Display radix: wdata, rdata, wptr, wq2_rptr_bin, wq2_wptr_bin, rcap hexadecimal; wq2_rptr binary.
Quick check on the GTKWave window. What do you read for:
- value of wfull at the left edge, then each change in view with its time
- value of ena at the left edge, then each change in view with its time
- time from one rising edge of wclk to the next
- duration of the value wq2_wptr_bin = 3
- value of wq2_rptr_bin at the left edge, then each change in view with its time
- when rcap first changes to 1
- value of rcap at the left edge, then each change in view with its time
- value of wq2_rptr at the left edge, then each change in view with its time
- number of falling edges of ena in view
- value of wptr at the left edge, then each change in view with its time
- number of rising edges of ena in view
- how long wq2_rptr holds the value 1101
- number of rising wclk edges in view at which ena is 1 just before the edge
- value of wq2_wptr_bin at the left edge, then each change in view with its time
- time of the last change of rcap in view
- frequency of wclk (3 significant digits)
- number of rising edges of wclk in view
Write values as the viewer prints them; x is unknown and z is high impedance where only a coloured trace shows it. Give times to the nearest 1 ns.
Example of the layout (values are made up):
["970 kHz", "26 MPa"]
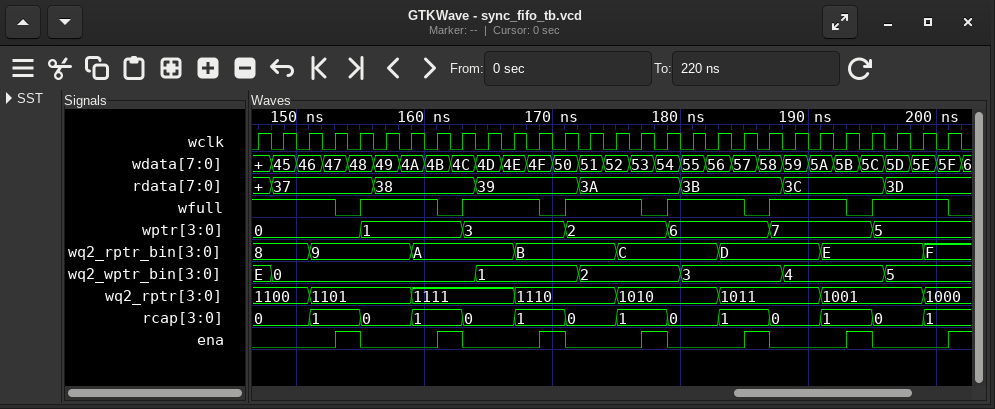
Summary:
["1, 0 at 153 ns, 1 at 155 ns, 0 at 161 ns, 1 at 163 ns, 0 at 169 ns, 1 at 171 ns, 0 at 177 ns, 1 at 179 ns, 0 at 185 ns, 1 at 187 ns, 0 at 193 ns, 1 at 195 ns, 0 at 201 ns", "0, 1 at 153 ns, 0 at 155 ns, 1 at 161 ns, 0 at 163 ns, 1 at 169 ns, 0 at 171 ns, 1 at 177 ns, 0 at 179 ns, 1 at 185 ns, 0 at 187 ns, 1 at 193 ns, 0 at 195 ns, 1 at 201 ns", "2 ns", "8 ns", "8, 9 at 151 ns, A at 159 ns, B at 167 ns, C at 175 ns, D at 183 ns, E at 191 ns, F at 199 ns", "151 ns", "0, 1 at 151 ns, 0 at 155 ns, 1 at 159 ns, 0 at 163 ns, 1 at 167 ns, 0 at 171 ns, 1 at 175 ns, 0 at 179 ns, 1 at 183 ns, 0 at 187 ns, 1 at 191 ns, 0 at 195 ns, 1 at 199 ns", "1100, 1101 at 151 ns, 1111 at 159 ns, 1110 at 167 ns, 1010 at 175 ns, 1011 at 183 ns, 1001 at 191 ns, 1000 at 199 ns", "6", "0, 1 at 155 ns, 3 at 163 ns, 2 at 171 ns, 6 at 179 ns, 7 at 187 ns, 5 at 195 ns", "7", "8 ns", "6", "E, 0 at 148 ns, 1 at 164 ns, 2 at 172 ns, 3 at 180 ns, 4 at 188 ns, 5 at 196 ns", "199 ns", "500 MHz", "28"]
